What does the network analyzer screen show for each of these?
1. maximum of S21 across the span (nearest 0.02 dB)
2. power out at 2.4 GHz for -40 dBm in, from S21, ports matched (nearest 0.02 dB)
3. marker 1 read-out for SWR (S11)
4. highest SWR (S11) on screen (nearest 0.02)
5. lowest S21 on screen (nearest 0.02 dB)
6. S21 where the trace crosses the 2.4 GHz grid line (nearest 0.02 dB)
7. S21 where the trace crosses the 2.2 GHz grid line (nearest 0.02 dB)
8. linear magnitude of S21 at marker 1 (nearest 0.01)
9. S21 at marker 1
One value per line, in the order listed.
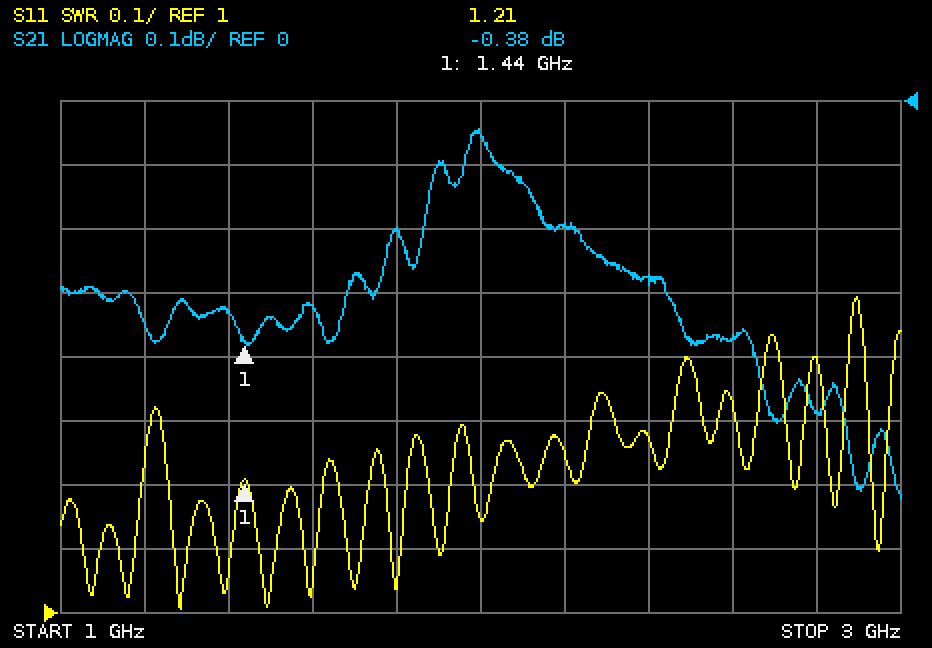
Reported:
-0.04 dB
-40.28 dBm
1.21
1.50
-0.62 dB
-0.28 dB
-0.20 dB
0.96
-0.38 dB
